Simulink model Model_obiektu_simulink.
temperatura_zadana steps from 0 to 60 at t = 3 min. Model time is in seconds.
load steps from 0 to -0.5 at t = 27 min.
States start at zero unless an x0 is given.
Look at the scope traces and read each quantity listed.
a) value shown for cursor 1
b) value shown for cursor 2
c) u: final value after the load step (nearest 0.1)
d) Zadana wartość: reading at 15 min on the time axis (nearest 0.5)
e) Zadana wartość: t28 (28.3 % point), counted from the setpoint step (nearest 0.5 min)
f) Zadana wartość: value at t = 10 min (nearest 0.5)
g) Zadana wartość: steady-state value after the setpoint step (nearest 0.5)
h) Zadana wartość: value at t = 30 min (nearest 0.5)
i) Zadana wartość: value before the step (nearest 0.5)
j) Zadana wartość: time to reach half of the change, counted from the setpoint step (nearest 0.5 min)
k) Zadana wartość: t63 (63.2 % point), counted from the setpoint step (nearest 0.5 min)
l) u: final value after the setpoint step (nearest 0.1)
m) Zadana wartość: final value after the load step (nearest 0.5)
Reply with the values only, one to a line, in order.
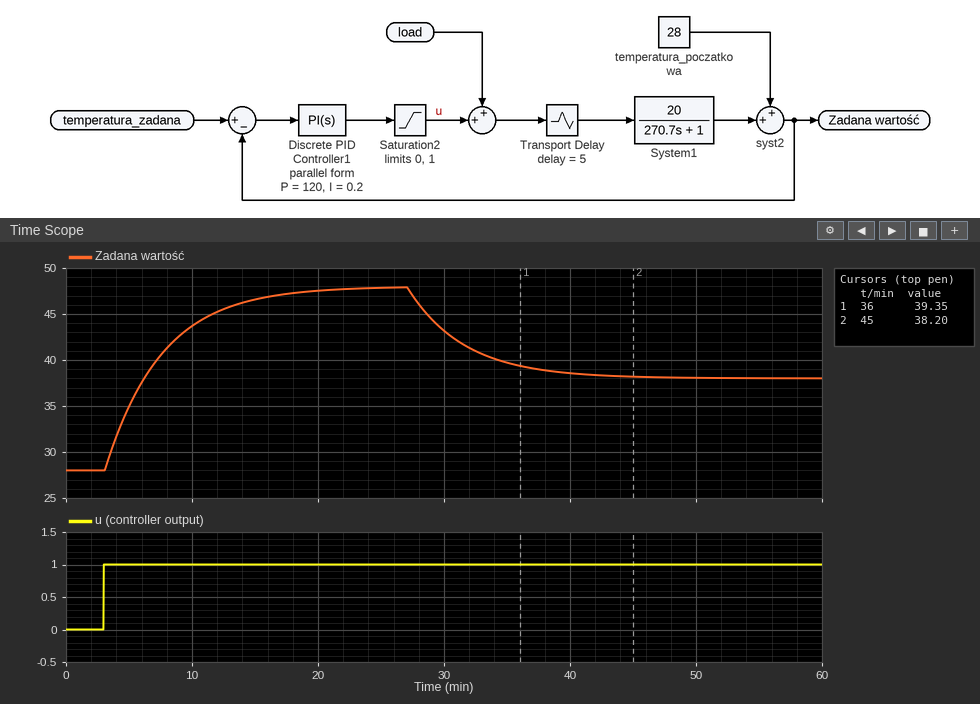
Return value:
39.35
38.20
1.0
46.5
1.5 min
43.5
48.0
43.0
28.0
3.0 min
4.5 min
1.0
38.0
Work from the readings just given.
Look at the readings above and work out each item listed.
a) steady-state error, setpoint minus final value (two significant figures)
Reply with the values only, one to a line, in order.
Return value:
12
